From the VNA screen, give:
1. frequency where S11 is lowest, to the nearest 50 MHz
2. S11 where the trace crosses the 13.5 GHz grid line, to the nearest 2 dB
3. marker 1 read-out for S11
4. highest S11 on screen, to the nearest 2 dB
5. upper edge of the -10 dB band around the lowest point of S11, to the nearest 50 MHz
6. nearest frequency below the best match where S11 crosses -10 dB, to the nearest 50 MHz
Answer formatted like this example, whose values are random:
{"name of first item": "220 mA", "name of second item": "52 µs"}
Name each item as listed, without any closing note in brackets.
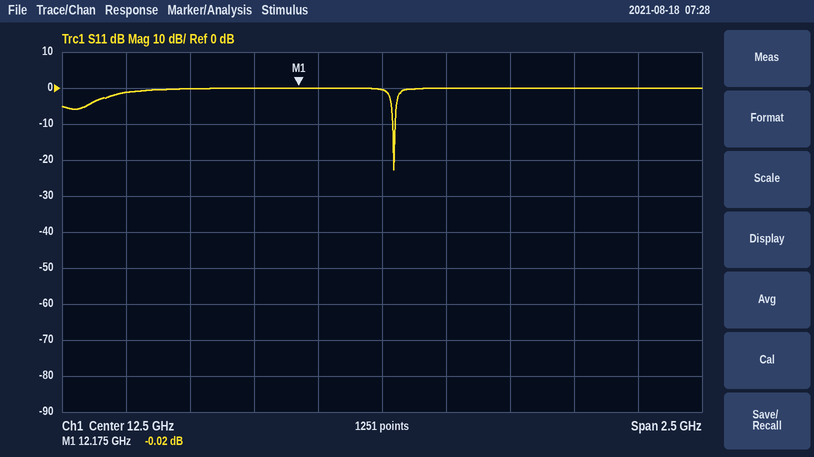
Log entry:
{"frequency where S11 is lowest, to the nearest 50 MHz": "12.55 GHz", "S11 where the trace crosses the 13.5 GHz grid line, to the nearest 2 dB": "0 dB", "marker 1 read-out for S11": "-0.02 dB", "highest S11 on screen, to the nearest 2 dB": "0 dB", "upper edge of the -10 dB band around the lowest point of S11, to the nearest 50 MHz": "12.55 GHz", "nearest frequency below the best match where S11 crosses -10 dB, to the nearest 50 MHz": "12.55 GHz"}
